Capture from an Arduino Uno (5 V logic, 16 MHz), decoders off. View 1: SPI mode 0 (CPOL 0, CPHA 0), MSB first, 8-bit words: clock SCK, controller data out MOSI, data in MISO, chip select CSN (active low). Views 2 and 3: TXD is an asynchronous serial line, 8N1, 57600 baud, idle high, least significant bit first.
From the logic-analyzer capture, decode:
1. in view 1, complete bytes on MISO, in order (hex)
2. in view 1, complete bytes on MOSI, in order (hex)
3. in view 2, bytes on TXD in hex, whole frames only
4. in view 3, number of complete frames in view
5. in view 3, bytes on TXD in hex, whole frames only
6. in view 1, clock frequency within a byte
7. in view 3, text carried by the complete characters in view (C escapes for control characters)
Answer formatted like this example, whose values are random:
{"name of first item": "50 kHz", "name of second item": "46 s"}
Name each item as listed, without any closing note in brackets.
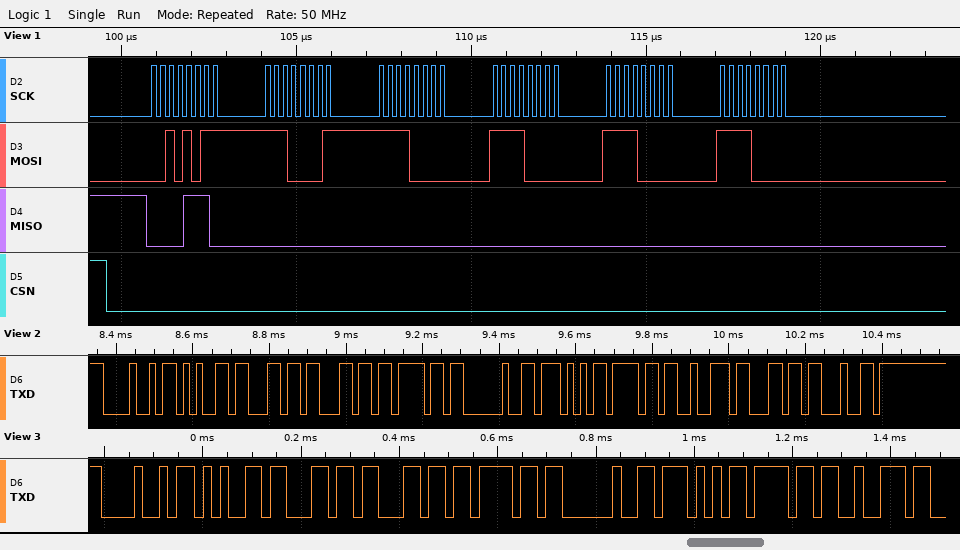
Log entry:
{"in view 1, complete bytes on MISO, in order": "0E 00 00 00 00 00", "in view 1, complete bytes on MOSI, in order": "2B E1 F0 F0 F0 F0", "in view 2, bytes on TXD in hex, whole frames only": "0x48 0x65 0x6C 0x6C 0x6F 0x20 0x57 0x6F 0x72 0x6C 0x64", "in view 3, number of complete frames in view": "9", "in view 3, bytes on TXD in hex, whole frames only": "48 65 6C 6C 6F 20 57 6F 72", "in view 1, clock frequency within a byte": "4 MHz", "in view 3, text carried by the complete characters in view": "\"Hello Wor\""}
